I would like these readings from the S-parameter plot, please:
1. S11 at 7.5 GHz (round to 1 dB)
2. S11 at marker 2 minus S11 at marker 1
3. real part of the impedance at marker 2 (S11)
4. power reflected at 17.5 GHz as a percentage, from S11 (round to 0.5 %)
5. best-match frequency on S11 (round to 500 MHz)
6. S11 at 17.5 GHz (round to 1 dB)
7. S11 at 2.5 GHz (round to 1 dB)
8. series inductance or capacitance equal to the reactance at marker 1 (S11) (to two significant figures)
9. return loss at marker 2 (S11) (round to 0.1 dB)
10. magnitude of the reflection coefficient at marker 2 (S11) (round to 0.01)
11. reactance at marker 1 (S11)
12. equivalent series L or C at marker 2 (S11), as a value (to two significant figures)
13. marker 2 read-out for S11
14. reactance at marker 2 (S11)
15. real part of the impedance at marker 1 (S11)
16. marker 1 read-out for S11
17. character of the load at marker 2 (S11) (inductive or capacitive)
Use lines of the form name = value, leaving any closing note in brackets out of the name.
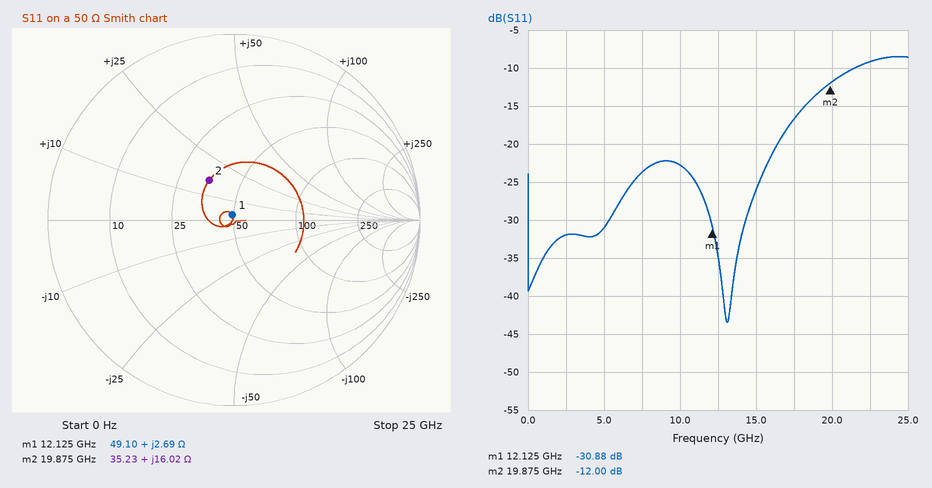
S11 at 7.5 GHz = -24 dB
S11 at marker 2 minus S11 at marker 1 = 18.88 dB
real part of the impedance at marker 2 = 35.23 Ω
power reflected at 17.5 GHz as a percentage, from S11 = 2.0 %
best-match frequency on S11 = 13.0 GHz
S11 at 17.5 GHz = -17 dB
S11 at 2.5 GHz = -32 dB
series inductance or capacitance equal to the reactance at marker 1 (S11) = 35 pH
return loss at marker 2 (S11) = 12.0 dB
magnitude of the reflection coefficient at marker 2 (S11) = 0.25
reactance at marker 1 = +2.69 Ω
equivalent series L or C at marker 2 (S11), as a value = 130 pH
marker 2 read-out for S11 = -12.00 dB
reactance at marker 2 = +16.02 Ω
real part of the impedance at marker 1 = 49.10 Ω
marker 1 read-out for S11 = -30.88 dB
character of the load at marker 2 (S11) = inductive
